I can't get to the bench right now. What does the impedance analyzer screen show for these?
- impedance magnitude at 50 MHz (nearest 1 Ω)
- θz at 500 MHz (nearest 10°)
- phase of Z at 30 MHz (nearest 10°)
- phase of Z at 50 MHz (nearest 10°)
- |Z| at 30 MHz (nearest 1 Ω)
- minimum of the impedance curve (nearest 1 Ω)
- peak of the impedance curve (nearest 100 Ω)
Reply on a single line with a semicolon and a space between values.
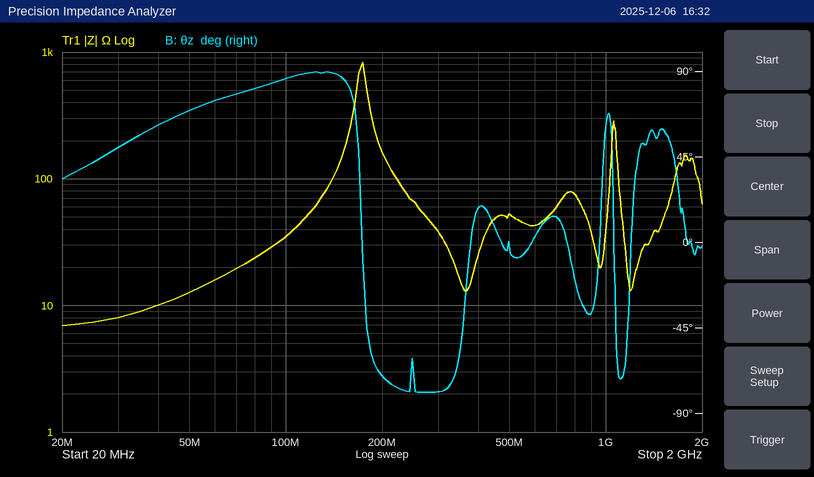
13 Ω; 0°; 50°; 70°; 8 Ω; 7 Ω; 800 Ω
